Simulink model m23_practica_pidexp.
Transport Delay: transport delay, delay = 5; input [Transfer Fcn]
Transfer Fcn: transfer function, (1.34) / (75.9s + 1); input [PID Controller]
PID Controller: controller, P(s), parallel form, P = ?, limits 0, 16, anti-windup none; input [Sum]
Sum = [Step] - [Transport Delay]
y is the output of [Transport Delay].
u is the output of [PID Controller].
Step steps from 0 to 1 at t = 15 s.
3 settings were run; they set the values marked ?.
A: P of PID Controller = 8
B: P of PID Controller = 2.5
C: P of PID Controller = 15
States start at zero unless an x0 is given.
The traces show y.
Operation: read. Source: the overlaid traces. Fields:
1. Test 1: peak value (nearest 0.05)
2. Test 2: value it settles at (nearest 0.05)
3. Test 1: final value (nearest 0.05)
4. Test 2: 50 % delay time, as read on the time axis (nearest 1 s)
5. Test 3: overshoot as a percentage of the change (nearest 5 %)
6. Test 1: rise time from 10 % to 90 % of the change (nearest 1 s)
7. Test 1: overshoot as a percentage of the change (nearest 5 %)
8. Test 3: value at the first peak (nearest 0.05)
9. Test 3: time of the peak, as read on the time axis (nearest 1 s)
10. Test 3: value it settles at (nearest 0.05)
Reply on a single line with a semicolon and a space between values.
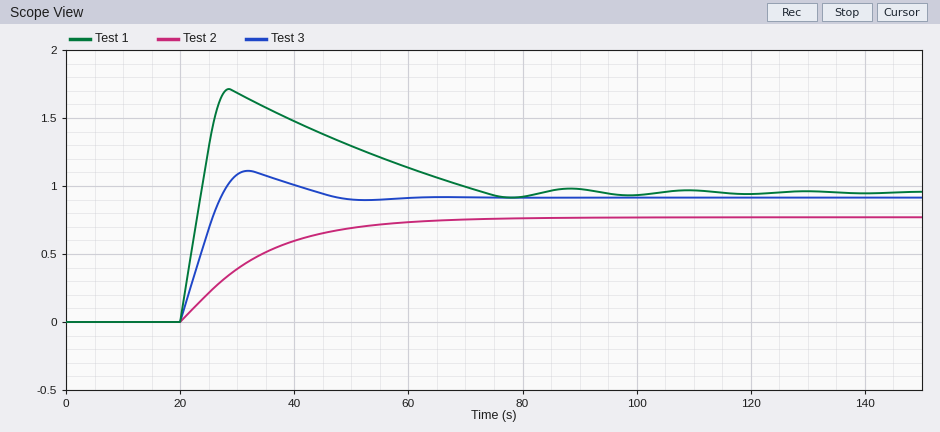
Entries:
1.70; 0.75; 0.95; 30 s; 20 %; 3 s; 80 %; 1.10; 32 s; 0.90
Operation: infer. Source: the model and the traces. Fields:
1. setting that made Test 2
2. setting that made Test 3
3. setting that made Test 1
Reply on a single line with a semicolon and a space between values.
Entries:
B; A; C
